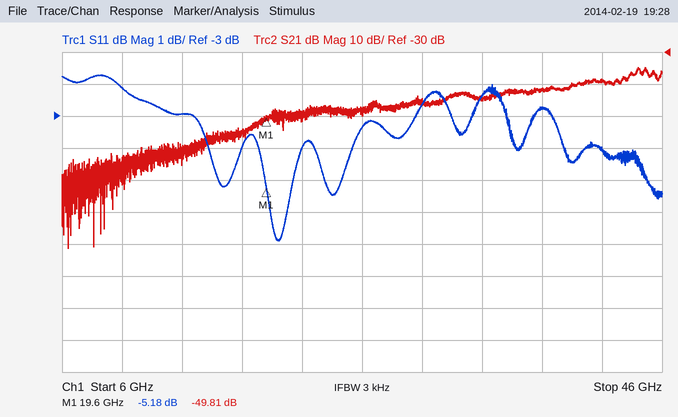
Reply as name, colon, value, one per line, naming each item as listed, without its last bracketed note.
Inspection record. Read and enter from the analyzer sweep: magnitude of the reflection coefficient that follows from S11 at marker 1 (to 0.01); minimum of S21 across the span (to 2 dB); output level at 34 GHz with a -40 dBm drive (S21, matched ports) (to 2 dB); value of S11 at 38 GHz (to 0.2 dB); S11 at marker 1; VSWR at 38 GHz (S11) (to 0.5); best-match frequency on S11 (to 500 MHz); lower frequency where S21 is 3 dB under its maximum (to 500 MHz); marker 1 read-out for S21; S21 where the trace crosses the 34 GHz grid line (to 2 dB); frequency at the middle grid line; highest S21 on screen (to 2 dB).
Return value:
magnitude of the reflection coefficient that follows from S11 at marker 1: 0.55
minimum of S21 across the span: -92 dB
output level at 34 GHz with a -40 dBm drive (S21, matched ports): -84 dBm
value of S11 at 38 GHz: -2.8 dB
S11 at marker 1: -5.18 dB
VSWR at 38 GHz (S11): 6.5
best-match frequency on S11: 20.5 GHz
lower frequency where S21 is 3 dB under its maximum: 44.0 GHz
marker 1 read-out for S21: -49.81 dB
S21 where the trace crosses the 34 GHz grid line: -44 dB
frequency at the middle grid line: 26 GHz
highest S21 on screen: -34 dB
